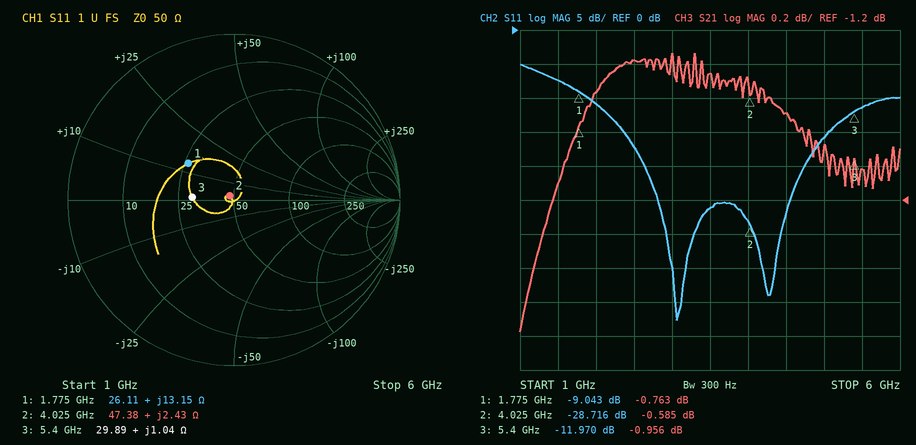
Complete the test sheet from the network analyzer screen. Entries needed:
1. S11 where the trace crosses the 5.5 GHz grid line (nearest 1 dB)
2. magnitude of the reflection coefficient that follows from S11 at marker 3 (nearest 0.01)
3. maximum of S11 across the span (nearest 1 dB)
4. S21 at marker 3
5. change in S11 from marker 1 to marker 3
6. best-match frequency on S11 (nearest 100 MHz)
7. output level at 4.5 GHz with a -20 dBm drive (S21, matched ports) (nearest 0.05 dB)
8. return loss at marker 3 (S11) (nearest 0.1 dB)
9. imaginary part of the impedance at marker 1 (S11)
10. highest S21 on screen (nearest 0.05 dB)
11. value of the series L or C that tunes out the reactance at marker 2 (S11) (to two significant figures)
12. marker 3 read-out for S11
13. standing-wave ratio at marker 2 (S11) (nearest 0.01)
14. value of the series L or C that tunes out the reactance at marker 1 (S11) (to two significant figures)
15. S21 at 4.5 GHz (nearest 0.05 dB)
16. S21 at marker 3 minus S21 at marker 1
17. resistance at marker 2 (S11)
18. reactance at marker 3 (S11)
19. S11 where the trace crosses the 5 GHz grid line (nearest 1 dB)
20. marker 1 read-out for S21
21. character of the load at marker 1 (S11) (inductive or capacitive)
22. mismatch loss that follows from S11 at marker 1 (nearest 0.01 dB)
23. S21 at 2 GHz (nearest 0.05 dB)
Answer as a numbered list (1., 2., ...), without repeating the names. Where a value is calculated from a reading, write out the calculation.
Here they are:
1. -11 dB
2. 10^(-11.97/20) ≈ 0.25
3. -5 dB
4. -0.956 dB
5. -11.97 − (-9.043) = -2.927 dB
6. 3.1 GHz
7. -20 dBm + (-0.70 dB) = -20.70 dBm
8. 12.0 dB
9. +13.15 Ω
10. -0.35 dB
11. C = 1/(2π × 4.025 GHz × 2.43 Ω) ≈ 16 pF
12. -11.970 dB
13. 1.08
14. C = 1/(2π × 1.775 GHz × 13.15 Ω) ≈ 6.8 pF
15. -0.70 dB
16. -0.956 − (-0.763) = -0.193 dB
17. 47.38 Ω
18. +1.04 Ω
19. -16 dB
20. -0.763 dB
21. inductive
22. −10 log10(1 − 10^(-9.043/10)) ≈ 0.58 dB
23. -0.55 dB
